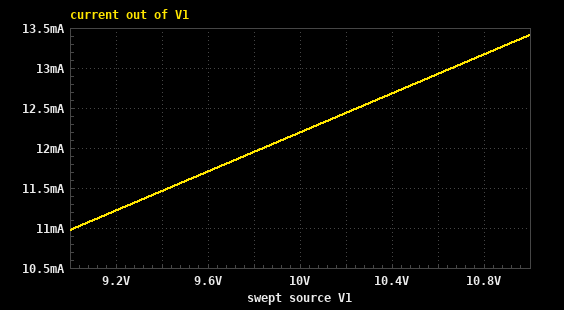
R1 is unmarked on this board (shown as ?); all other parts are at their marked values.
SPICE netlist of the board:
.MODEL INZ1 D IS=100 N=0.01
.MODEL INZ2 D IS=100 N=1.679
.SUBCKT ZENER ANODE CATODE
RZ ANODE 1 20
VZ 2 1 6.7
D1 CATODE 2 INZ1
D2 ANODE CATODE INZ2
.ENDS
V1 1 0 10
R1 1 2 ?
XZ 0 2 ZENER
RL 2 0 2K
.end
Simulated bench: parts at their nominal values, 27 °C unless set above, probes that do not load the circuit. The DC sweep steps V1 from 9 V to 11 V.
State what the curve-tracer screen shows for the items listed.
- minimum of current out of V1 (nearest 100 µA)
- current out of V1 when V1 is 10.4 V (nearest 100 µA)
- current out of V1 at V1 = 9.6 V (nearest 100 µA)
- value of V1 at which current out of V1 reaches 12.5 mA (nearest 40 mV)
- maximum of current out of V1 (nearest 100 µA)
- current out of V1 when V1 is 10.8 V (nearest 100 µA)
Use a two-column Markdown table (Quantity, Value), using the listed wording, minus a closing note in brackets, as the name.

| Quantity | Value |
|---|---|
| minimum of current out of V1 | 11.0 mA |
| current out of V1 when V1 is 10.4 V | 12.7 mA |
| current out of V1 at V1 = 9.6 V | 11.7 mA |
| value of V1 at which current out of V1 reaches 12.5 mA | 10.24 V |
| maximum of current out of V1 | 13.4 mA |
| current out of V1 when V1 is 10.8 V | 13.2 mA |
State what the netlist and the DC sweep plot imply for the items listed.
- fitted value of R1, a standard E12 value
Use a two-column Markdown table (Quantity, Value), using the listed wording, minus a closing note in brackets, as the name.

| Quantity | Value |
|---|---|
| fitted value of R1, a standard E12 value | 820 Ω |
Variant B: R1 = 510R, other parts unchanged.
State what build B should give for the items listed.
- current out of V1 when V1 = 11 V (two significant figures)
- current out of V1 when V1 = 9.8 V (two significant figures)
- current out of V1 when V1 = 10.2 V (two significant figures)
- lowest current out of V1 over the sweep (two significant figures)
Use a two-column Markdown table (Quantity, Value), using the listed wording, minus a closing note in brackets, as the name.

| Quantity | Value |
|---|---|
| current out of V1 when V1 = 11 V | 22 mA |
| current out of V1 when V1 = 9.8 V | 19 mA |
| current out of V1 when V1 = 10.2 V | 20 mA |
| lowest current out of V1 over the sweep | 18 mA |
